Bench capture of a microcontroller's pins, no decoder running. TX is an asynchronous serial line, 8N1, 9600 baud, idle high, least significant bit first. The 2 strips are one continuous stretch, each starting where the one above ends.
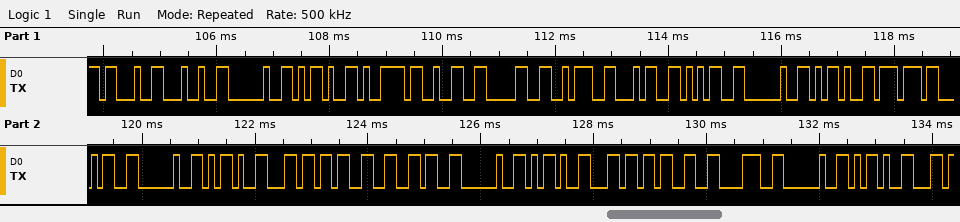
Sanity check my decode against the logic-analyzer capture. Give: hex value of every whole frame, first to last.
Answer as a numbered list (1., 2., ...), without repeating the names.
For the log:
1. 23 24 20 2D 79 32 30 3A 34 35 20 2D 77 34 20 2D 6C 33 36 20 2D 6C 33 38 20 2D
